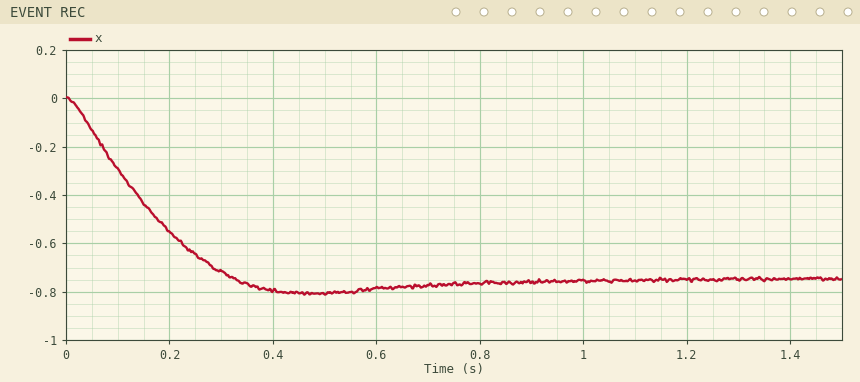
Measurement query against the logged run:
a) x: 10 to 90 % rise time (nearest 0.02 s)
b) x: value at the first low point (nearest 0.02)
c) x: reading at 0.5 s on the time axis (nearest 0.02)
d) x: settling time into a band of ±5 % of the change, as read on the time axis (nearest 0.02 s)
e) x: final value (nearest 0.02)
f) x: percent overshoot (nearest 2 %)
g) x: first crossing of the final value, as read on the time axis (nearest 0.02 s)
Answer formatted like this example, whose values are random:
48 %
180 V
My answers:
0.24 s
-0.80
-0.80
0.64 s
-0.74
8 %
0.32 s
